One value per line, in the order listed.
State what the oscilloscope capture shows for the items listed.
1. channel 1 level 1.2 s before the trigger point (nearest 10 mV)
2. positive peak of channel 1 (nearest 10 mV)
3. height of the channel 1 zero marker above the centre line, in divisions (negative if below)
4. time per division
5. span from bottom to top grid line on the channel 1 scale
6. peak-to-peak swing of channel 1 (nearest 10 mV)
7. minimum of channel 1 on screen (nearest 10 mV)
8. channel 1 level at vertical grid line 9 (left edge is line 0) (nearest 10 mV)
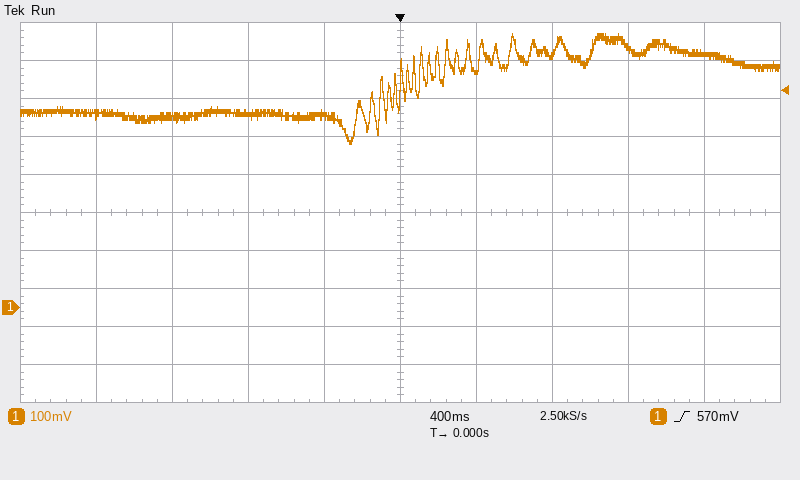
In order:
500 mV
720 mV
-2.5 div
400 ms
1 V
290 mV
430 mV
670 mV
